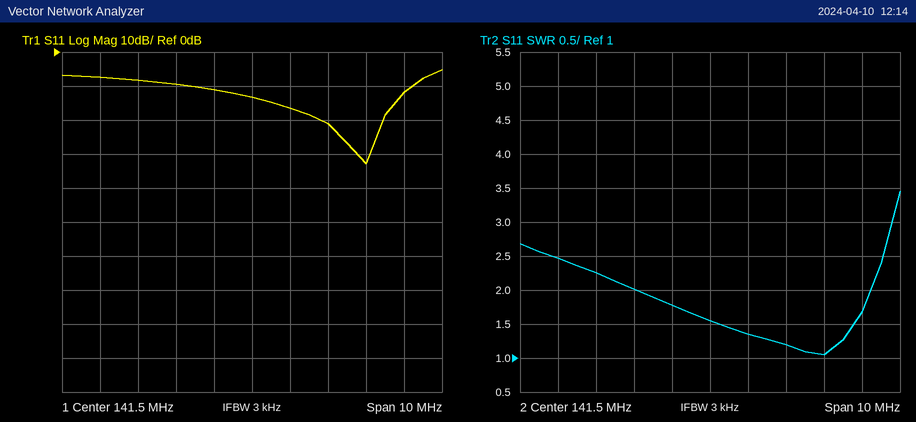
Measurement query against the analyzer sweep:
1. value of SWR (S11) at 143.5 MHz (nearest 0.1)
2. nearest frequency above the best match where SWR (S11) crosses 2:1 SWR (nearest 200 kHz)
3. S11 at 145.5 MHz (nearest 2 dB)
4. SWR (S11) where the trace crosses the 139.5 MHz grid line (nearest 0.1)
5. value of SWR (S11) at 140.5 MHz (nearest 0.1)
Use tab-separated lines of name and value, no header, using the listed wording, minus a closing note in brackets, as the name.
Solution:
value of SWR (S11) at 143.5 MHz	1.2
nearest frequency above the best match where SWR (S11) crosses 2:1 SWR	145.8 MHz
S11 at 145.5 MHz	-12 dB
SWR (S11) where the trace crosses the 139.5 MHz grid line	2.0
value of SWR (S11) at 140.5 MHz	1.8
